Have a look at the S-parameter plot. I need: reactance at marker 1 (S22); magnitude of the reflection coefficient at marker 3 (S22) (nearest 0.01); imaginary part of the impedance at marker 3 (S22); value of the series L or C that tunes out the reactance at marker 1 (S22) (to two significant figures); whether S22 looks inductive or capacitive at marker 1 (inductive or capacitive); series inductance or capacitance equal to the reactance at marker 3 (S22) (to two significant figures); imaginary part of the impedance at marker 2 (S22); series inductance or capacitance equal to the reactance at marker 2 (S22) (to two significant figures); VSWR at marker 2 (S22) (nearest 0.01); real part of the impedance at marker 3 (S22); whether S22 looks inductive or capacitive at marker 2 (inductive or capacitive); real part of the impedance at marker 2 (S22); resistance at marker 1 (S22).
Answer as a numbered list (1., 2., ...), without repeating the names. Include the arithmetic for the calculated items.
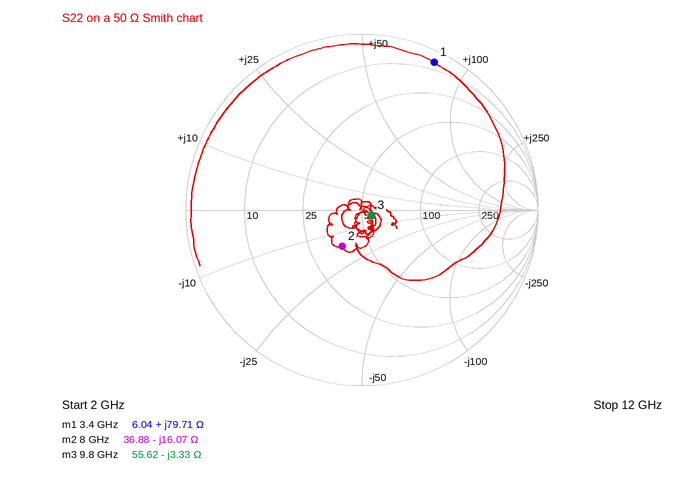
1. +79.71 Ω
2. 0.06
3. -3.33 Ω
4. C = 1/(2π × 3.4 GHz × 79.71 Ω) ≈ 587 fF, so 590 fF to two significant figures
5. inductive
6. C = 1/(2π × 9.8 GHz × 3.33 Ω) ≈ 4.9 pF
7. -16.07 Ω
8. C = 1/(2π × 8 GHz × 16.07 Ω) ≈ 1.2 pF
9. 1.61
10. 55.62 Ω
11. capacitive
12. 36.88 Ω
13. 6.04 Ω
